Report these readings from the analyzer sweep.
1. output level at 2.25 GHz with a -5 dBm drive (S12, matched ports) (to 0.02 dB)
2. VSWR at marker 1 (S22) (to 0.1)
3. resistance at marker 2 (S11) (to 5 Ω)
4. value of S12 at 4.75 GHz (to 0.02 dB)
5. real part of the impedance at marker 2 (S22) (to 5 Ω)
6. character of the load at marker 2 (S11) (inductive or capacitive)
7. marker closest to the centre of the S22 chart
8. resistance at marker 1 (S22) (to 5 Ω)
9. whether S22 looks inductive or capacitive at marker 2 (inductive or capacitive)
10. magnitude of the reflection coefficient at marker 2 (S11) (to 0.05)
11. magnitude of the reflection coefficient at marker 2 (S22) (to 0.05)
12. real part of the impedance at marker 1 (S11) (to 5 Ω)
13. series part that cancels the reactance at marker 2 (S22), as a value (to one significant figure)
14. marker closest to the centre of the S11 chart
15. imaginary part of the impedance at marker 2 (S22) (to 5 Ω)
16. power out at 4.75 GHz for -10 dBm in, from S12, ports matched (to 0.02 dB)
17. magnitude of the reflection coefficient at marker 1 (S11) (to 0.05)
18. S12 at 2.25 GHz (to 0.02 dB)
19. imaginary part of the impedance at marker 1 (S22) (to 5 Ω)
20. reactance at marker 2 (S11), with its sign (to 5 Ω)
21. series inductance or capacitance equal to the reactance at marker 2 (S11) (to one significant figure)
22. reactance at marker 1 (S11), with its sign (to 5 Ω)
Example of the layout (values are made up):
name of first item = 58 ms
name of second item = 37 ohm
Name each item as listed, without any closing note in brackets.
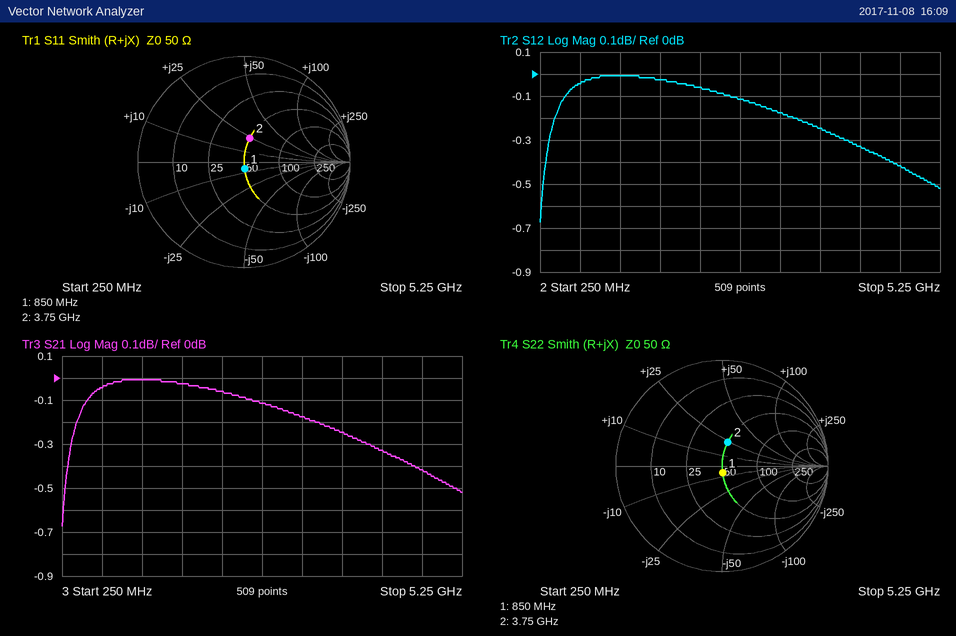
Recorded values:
output level at 2.25 GHz with a -5 dBm drive (S12, matched ports) = -5.06 dBm
VSWR at marker 1 (S22) = 1.1
resistance at marker 2 (S11) = 50 Ω
value of S12 at 4.75 GHz = -0.42 dB
real part of the impedance at marker 2 (S22) = 50 Ω
character of the load at marker 2 (S11) = inductive
marker closest to the centre of the S22 chart = marker 1
resistance at marker 1 (S22) = 50 Ω
whether S22 looks inductive or capacitive at marker 2 = inductive
magnitude of the reflection coefficient at marker 2 (S11) = 0.25
magnitude of the reflection coefficient at marker 2 (S22) = 0.25
real part of the impedance at marker 1 (S11) = 50 Ω
series part that cancels the reactance at marker 2 (S22), as a value = 2 pF
marker closest to the centre of the S11 chart = marker 1
imaginary part of the impedance at marker 2 (S22) = +25 Ω
power out at 4.75 GHz for -10 dBm in, from S12, ports matched = -10.42 dBm
magnitude of the reflection coefficient at marker 1 (S11) = 0.05
S12 at 2.25 GHz = -0.06 dB
imaginary part of the impedance at marker 1 (S22) = -5 Ω
reactance at marker 2 (S11), with its sign = +25 Ω
series inductance or capacitance equal to the reactance at marker 2 (S11) = 1 nH
reactance at marker 1 (S11), with its sign = -5 Ω
